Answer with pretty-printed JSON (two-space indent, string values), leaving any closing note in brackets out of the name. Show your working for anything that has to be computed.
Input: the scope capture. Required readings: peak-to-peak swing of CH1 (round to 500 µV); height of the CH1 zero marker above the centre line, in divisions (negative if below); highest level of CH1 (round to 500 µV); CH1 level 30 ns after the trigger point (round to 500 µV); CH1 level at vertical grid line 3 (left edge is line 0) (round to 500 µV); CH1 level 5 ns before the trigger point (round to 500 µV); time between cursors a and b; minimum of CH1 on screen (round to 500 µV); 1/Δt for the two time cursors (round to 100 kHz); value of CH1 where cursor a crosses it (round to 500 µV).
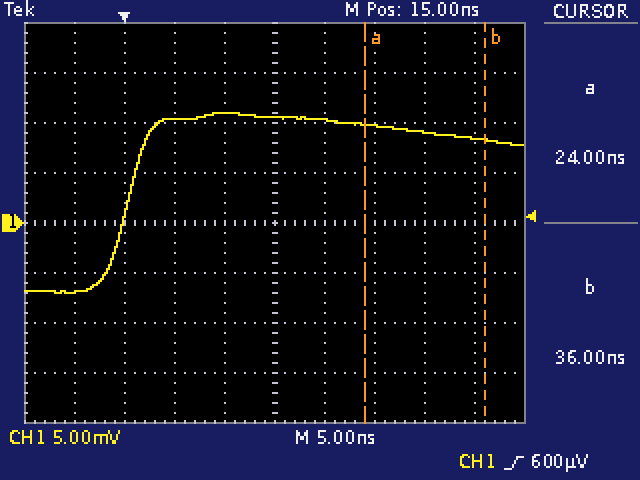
{
  "peak-to-peak swing of CH1": "11.0 mV − (-7.0 mV) = 18.0 mV",
  "height of the CH1 zero marker above the centre line, in divisions": "0.0 div",
  "highest level of CH1": "11.0 mV",
  "CH1 level 30 ns after the trigger point": "9.0 mV",
  "CH1 level at vertical grid line 3 (left edge is line 0)": "10.5 mV",
  "CH1 level 5 ns before the trigger point": "-7.0 mV",
  "time between cursors a and b": "36 ns − (24 ns) = 12.0 ns",
  "minimum of CH1 on screen": "-7.0 mV",
  "1/Δt for the two time cursors": "1 / 12.0 ns ≈ 83.3 MHz",
  "value of CH1 where cursor a crosses it": "10.0 mV"
}
